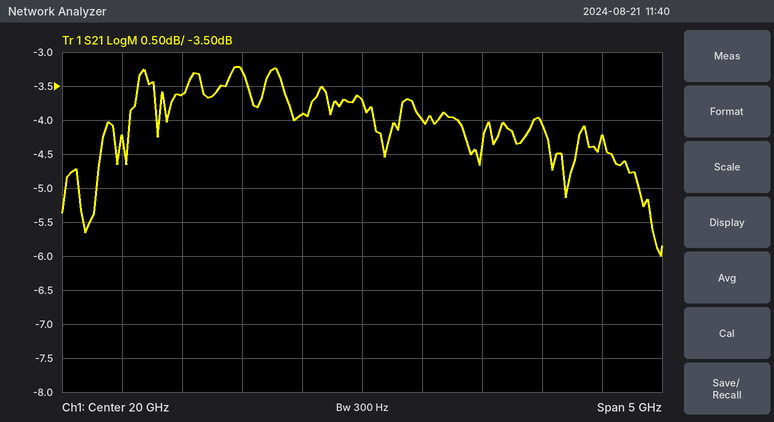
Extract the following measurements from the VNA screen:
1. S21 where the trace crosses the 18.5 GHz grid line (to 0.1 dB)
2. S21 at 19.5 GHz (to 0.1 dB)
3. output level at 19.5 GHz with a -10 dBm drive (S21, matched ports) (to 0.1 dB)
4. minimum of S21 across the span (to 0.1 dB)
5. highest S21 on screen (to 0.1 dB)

-3.6 dB
-3.9 dB
-13.9 dBm
-6.0 dB
-3.2 dB
